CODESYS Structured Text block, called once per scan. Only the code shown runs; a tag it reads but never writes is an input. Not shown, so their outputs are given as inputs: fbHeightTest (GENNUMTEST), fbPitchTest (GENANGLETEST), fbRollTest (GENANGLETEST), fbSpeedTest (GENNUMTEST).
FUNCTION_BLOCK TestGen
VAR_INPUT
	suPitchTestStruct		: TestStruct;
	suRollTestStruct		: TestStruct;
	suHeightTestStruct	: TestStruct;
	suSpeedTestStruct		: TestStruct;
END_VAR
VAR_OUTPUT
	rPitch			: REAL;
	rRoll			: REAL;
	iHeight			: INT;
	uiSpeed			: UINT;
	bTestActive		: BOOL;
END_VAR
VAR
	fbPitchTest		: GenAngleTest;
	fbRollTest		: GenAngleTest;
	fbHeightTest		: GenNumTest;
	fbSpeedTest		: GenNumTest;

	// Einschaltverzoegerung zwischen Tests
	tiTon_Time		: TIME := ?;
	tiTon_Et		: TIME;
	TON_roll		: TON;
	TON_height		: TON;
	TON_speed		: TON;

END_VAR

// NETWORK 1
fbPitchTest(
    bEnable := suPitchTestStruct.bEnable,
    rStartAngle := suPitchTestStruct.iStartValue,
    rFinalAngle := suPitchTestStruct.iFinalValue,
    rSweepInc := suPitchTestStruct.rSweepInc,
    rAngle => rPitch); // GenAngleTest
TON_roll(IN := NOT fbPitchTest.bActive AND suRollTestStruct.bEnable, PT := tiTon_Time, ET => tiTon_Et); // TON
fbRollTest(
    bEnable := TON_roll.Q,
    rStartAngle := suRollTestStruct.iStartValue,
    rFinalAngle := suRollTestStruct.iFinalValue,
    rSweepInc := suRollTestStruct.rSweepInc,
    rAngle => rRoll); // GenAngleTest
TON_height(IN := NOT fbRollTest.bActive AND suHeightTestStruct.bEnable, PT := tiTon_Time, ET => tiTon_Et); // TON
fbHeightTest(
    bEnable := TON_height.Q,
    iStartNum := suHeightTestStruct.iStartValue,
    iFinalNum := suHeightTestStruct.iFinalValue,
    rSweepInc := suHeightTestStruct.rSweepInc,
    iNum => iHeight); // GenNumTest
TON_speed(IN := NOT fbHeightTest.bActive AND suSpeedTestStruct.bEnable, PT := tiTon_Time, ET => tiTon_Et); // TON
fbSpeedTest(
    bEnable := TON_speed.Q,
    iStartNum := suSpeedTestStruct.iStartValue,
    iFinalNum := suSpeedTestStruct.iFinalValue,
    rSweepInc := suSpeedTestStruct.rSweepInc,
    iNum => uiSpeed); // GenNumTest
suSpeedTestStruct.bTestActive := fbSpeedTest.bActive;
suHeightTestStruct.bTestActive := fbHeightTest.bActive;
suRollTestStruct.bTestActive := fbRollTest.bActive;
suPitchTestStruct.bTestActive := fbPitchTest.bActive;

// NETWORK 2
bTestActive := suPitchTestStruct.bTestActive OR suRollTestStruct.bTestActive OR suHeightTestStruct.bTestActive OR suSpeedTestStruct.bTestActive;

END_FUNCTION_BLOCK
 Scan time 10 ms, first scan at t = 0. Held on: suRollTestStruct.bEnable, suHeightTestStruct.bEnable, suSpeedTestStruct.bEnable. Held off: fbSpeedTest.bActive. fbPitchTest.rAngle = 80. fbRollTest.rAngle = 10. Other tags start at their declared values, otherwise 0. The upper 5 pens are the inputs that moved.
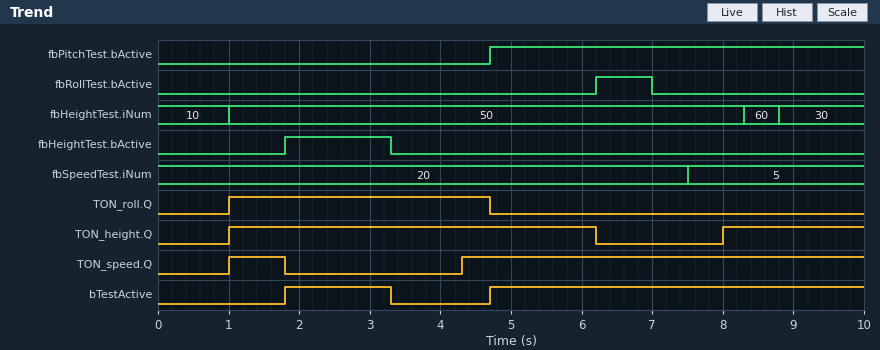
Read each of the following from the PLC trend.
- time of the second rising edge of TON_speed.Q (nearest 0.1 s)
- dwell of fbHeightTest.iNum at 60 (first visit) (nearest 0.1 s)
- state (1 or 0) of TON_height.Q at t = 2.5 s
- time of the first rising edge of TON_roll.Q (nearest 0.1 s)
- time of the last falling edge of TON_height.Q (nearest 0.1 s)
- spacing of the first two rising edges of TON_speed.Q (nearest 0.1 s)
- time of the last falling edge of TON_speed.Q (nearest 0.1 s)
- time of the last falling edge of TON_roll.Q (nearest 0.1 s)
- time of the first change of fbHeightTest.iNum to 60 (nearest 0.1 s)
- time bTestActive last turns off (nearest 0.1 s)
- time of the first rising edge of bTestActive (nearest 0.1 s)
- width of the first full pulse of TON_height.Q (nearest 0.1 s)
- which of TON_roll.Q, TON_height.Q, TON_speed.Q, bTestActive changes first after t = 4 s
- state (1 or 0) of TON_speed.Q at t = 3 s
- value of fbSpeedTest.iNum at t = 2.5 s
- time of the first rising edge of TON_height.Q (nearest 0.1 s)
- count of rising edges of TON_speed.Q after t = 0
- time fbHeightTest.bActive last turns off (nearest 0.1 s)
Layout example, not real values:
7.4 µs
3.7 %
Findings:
4.3 s
0.5 s
1
1.0 s
6.2 s
3.3 s
1.8 s
4.7 s
8.3 s
3.3 s
1.8 s
5.2 s
TON_speed.Q
0
20
1.0 s
2
3.3 s
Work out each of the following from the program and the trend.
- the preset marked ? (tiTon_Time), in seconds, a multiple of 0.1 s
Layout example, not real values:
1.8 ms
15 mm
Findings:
1.0 s
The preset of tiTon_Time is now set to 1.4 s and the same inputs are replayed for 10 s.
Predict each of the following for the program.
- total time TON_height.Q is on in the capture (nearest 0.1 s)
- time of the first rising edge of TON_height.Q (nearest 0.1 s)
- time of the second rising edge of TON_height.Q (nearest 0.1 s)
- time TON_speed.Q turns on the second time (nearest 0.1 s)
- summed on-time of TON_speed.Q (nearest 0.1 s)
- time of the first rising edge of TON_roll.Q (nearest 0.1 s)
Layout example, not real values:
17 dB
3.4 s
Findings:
6.4 s
1.4 s
8.4 s
4.7 s
5.7 s
1.4 s
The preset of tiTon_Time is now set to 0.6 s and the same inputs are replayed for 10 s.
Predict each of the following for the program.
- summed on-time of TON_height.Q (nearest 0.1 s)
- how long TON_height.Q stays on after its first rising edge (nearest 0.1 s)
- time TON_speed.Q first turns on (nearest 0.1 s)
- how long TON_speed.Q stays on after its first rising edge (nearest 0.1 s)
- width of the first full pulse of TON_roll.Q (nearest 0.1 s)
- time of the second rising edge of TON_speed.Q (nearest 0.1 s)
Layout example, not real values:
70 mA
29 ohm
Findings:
8.0 s
5.6 s
0.6 s
1.2 s
4.1 s
3.9 s
